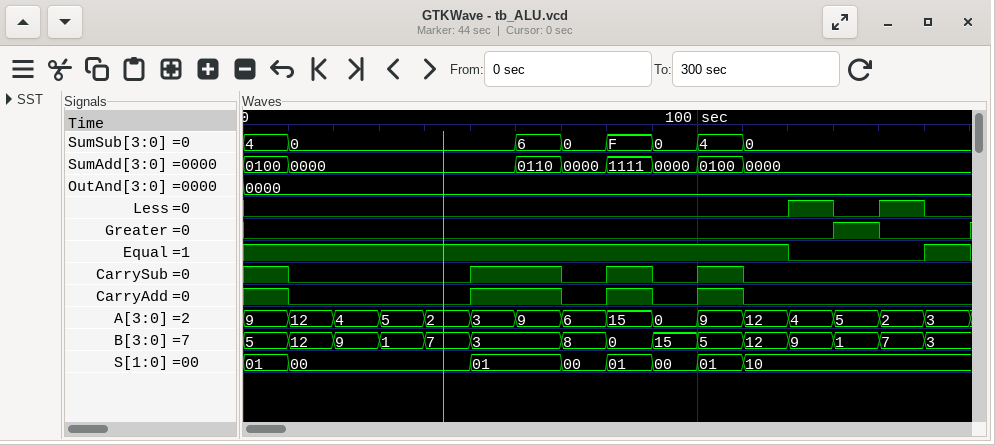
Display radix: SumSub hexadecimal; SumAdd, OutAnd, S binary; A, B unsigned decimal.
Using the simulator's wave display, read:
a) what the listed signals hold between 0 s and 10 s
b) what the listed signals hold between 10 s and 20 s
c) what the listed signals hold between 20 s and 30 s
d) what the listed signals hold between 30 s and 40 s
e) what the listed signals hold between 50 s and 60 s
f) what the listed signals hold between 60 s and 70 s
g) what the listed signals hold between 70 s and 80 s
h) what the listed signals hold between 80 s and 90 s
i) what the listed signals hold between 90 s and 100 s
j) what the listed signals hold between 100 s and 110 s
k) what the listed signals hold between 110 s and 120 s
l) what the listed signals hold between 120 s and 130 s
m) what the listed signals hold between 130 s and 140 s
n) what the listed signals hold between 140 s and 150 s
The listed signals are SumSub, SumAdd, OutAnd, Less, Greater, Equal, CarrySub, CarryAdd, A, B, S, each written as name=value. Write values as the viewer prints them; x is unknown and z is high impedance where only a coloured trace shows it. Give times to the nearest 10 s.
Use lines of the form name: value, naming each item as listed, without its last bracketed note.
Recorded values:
what the listed signals hold between 0 s and 10 s: SumSub=4, SumAdd=0100, OutAnd=0000, Less=0, Greater=0, Equal=1, CarrySub=1, CarryAdd=1, A=9, B=5, S=01
what the listed signals hold between 10 s and 20 s: SumSub=0, SumAdd=0000, OutAnd=0000, Less=0, Greater=0, Equal=1, CarrySub=0, CarryAdd=0, A=12, B=12, S=00
what the listed signals hold between 20 s and 30 s: SumSub=0, SumAdd=0000, OutAnd=0000, Less=0, Greater=0, Equal=1, CarrySub=0, CarryAdd=0, A=4, B=9, S=00
what the listed signals hold between 30 s and 40 s: SumSub=0, SumAdd=0000, OutAnd=0000, Less=0, Greater=0, Equal=1, CarrySub=0, CarryAdd=0, A=5, B=1, S=00
what the listed signals hold between 50 s and 60 s: SumSub=0, SumAdd=0000, OutAnd=0000, Less=0, Greater=0, Equal=1, CarrySub=1, CarryAdd=1, A=3, B=3, S=01
what the listed signals hold between 60 s and 70 s: SumSub=6, SumAdd=0110, OutAnd=0000, Less=0, Greater=0, Equal=1, CarrySub=1, CarryAdd=1, A=9, B=3, S=01
what the listed signals hold between 70 s and 80 s: SumSub=0, SumAdd=0000, OutAnd=0000, Less=0, Greater=0, Equal=1, CarrySub=0, CarryAdd=0, A=6, B=8, S=00
what the listed signals hold between 80 s and 90 s: SumSub=F, SumAdd=1111, OutAnd=0000, Less=0, Greater=0, Equal=1, CarrySub=1, CarryAdd=1, A=15, B=0, S=01
what the listed signals hold between 90 s and 100 s: SumSub=0, SumAdd=0000, OutAnd=0000, Less=0, Greater=0, Equal=1, CarrySub=0, CarryAdd=0, A=0, B=15, S=00
what the listed signals hold between 100 s and 110 s: SumSub=4, SumAdd=0100, OutAnd=0000, Less=0, Greater=0, Equal=1, CarrySub=1, CarryAdd=1, A=9, B=5, S=01
what the listed signals hold between 110 s and 120 s: SumSub=0, SumAdd=0000, OutAnd=0000, Less=0, Greater=0, Equal=1, CarrySub=0, CarryAdd=0, A=12, B=12, S=10
what the listed signals hold between 120 s and 130 s: SumSub=0, SumAdd=0000, OutAnd=0000, Less=1, Greater=0, Equal=0, CarrySub=0, CarryAdd=0, A=4, B=9, S=10
what the listed signals hold between 130 s and 140 s: SumSub=0, SumAdd=0000, OutAnd=0000, Less=0, Greater=1, Equal=0, CarrySub=0, CarryAdd=0, A=5, B=1, S=10
what the listed signals hold between 140 s and 150 s: SumSub=0, SumAdd=0000, OutAnd=0000, Less=1, Greater=0, Equal=0, CarrySub=0, CarryAdd=0, A=2, B=7, S=10
